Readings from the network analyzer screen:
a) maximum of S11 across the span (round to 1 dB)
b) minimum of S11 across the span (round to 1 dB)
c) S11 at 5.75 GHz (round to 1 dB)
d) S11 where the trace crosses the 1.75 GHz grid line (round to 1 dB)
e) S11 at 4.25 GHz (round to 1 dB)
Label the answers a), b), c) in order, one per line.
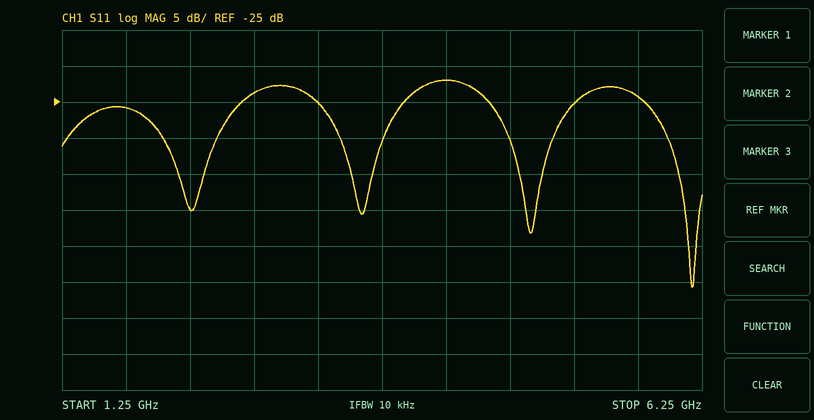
a) -22 dB
b) -51 dB
c) -24 dB
d) -26 dB
e) -22 dB
